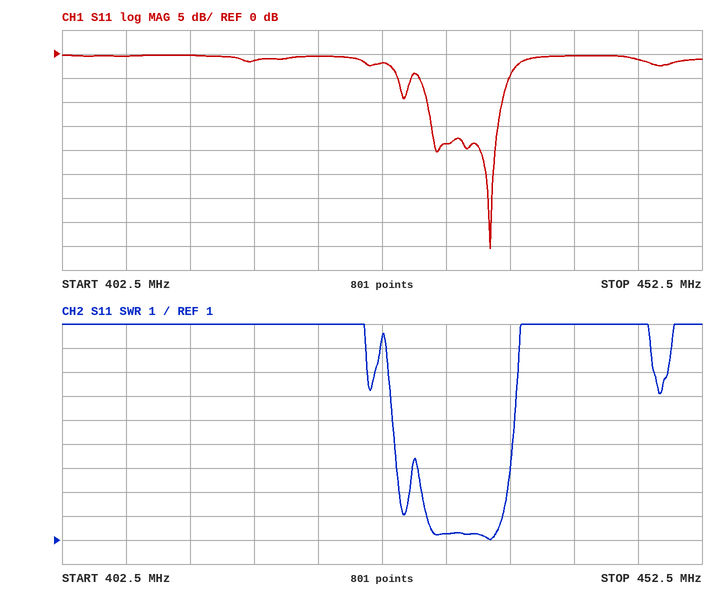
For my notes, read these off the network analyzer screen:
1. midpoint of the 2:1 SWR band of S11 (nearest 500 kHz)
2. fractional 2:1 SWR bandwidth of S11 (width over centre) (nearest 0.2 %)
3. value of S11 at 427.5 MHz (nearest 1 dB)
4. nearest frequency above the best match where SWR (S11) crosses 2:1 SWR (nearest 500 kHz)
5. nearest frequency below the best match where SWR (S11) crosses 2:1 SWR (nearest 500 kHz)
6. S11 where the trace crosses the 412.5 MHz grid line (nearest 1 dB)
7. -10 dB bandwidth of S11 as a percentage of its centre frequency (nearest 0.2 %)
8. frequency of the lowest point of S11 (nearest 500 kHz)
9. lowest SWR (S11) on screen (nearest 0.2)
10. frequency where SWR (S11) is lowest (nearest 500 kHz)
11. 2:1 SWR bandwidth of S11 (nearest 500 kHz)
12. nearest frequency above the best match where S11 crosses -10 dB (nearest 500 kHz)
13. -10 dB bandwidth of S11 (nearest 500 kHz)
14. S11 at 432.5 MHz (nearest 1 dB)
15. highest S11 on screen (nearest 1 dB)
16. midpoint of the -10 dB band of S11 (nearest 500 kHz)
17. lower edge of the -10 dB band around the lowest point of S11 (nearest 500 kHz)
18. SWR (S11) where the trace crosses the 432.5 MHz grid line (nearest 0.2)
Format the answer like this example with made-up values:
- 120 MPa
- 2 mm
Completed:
- 434.0 MHz
- 1.4 %
- -2 dB
- 437.0 MHz
- 431.0 MHz
- 0 dB
- 1.4 %
- 436.0 MHz
- 1.0
- 436.0 MHz
- 6.0 MHz
- 437.0 MHz
- 6.0 MHz
- -19 dB
- 0 dB
- 434.0 MHz
- 431.0 MHz
- 1.2
